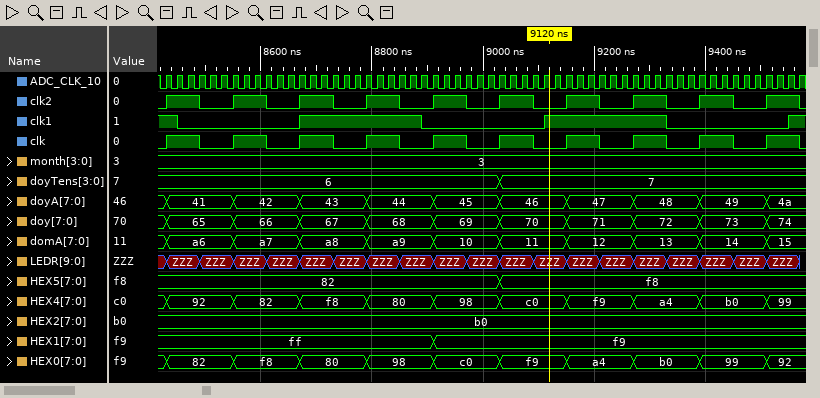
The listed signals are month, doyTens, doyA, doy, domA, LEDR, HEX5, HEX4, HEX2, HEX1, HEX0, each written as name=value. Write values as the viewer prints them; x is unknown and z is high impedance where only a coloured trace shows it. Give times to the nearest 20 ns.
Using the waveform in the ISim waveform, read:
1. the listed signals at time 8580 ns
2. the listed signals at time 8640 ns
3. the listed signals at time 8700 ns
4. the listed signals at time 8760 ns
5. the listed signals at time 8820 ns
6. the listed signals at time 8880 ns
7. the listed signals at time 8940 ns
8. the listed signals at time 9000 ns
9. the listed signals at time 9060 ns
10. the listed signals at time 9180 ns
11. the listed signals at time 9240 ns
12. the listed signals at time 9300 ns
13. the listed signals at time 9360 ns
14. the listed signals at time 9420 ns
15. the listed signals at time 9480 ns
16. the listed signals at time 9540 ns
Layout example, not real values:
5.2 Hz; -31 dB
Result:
month=3, doyTens=6, doyA=42, doy=66, domA=a7, LEDR=ZZZ, HEX5=82, HEX4=82, HEX2=b0, HEX1=ff, HEX0=f8; month=3, doyTens=6, doyA=42, doy=66, domA=a7, LEDR=ZZZ, HEX5=82, HEX4=82, HEX2=b0, HEX1=ff, HEX0=f8; month=3, doyTens=6, doyA=43, doy=67, domA=a8, LEDR=ZZZ, HEX5=82, HEX4=f8, HEX2=b0, HEX1=ff, HEX0=80; month=3, doyTens=6, doyA=43, doy=67, domA=a8, LEDR=ZZZ, HEX5=82, HEX4=f8, HEX2=b0, HEX1=ff, HEX0=80; month=3, doyTens=6, doyA=44, doy=68, domA=a9, LEDR=ZZZ, HEX5=82, HEX4=80, HEX2=b0, HEX1=ff, HEX0=98; month=3, doyTens=6, doyA=44, doy=68, domA=a9, LEDR=ZZZ, HEX5=82, HEX4=80, HEX2=b0, HEX1=ff, HEX0=98; month=3, doyTens=6, doyA=45, doy=69, domA=10, LEDR=ZZZ, HEX5=82, HEX4=98, HEX2=b0, HEX1=f9, HEX0=c0; month=3, doyTens=6, doyA=45, doy=69, domA=10, LEDR=ZZZ, HEX5=82, HEX4=98, HEX2=b0, HEX1=f9, HEX0=c0; month=3, doyTens=7, doyA=46, doy=70, domA=11, LEDR=ZZZ, HEX5=f8, HEX4=c0, HEX2=b0, HEX1=f9, HEX0=f9; month=3, doyTens=7, doyA=47, doy=71, domA=12, LEDR=ZZZ, HEX5=f8, HEX4=f9, HEX2=b0, HEX1=f9, HEX0=a4; month=3, doyTens=7, doyA=47, doy=71, domA=12, LEDR=ZZZ, HEX5=f8, HEX4=f9, HEX2=b0, HEX1=f9, HEX0=a4; month=3, doyTens=7, doyA=48, doy=72, domA=13, LEDR=ZZZ, HEX5=f8, HEX4=a4, HEX2=b0, HEX1=f9, HEX0=b0; month=3, doyTens=7, doyA=48, doy=72, domA=13, LEDR=ZZZ, HEX5=f8, HEX4=a4, HEX2=b0, HEX1=f9, HEX0=b0; month=3, doyTens=7, doyA=49, doy=73, domA=14, LEDR=ZZZ, HEX5=f8, HEX4=b0, HEX2=b0, HEX1=f9, HEX0=99; month=3, doyTens=7, doyA=49, doy=73, domA=14, LEDR=ZZZ, HEX5=f8, HEX4=b0, HEX2=b0, HEX1=f9, HEX0=99; month=3, doyTens=7, doyA=4a, doy=74, domA=15, LEDR=ZZZ, HEX5=f8, HEX4=99, HEX2=b0, HEX1=f9, HEX0=92
